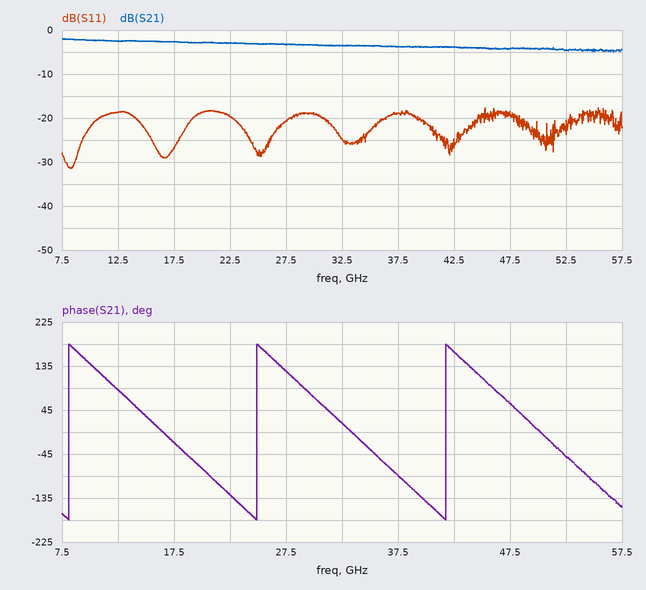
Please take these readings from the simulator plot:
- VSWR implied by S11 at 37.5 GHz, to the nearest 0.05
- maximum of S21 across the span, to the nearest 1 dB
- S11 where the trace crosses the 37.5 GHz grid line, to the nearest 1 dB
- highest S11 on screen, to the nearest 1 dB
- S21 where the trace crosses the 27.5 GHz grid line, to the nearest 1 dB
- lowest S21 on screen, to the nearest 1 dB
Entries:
1.25
-2 dB
-19 dB
-18 dB
-3 dB
-5 dB
